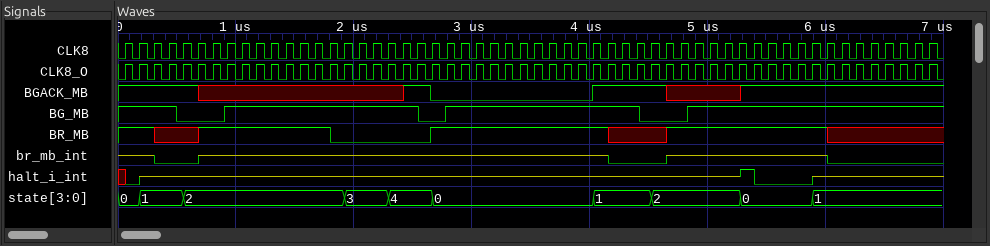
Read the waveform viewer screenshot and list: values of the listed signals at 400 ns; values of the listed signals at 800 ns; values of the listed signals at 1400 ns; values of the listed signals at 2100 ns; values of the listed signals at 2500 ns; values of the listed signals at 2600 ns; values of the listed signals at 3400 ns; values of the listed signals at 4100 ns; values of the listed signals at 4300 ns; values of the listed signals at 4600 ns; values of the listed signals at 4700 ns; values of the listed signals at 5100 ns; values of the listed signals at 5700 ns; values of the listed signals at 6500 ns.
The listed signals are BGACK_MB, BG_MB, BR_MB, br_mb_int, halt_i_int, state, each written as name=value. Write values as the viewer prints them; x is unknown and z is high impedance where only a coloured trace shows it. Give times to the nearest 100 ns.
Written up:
BGACK_MB=1, BG_MB=1, BR_MB=x, br_mb_int=0, halt_i_int=z, state=1
BGACK_MB=x, BG_MB=0, BR_MB=1, br_mb_int=z, halt_i_int=z, state=2
BGACK_MB=x, BG_MB=1, BR_MB=1, br_mb_int=z, halt_i_int=z, state=2
BGACK_MB=x, BG_MB=1, BR_MB=0, br_mb_int=z, halt_i_int=z, state=3
BGACK_MB=1, BG_MB=1, BR_MB=0, br_mb_int=z, halt_i_int=z, state=4
BGACK_MB=1, BG_MB=0, BR_MB=0, br_mb_int=z, halt_i_int=z, state=4
BGACK_MB=0, BG_MB=1, BR_MB=1, br_mb_int=z, halt_i_int=z, state=0
BGACK_MB=1, BG_MB=1, BR_MB=1, br_mb_int=z, halt_i_int=z, state=1
BGACK_MB=1, BG_MB=1, BR_MB=x, br_mb_int=0, halt_i_int=z, state=1
BGACK_MB=1, BG_MB=0, BR_MB=x, br_mb_int=0, halt_i_int=z, state=2
BGACK_MB=x, BG_MB=0, BR_MB=1, br_mb_int=z, halt_i_int=z, state=2
BGACK_MB=x, BG_MB=1, BR_MB=1, br_mb_int=z, halt_i_int=z, state=2
BGACK_MB=1, BG_MB=1, BR_MB=1, br_mb_int=z, halt_i_int=0, state=0
BGACK_MB=1, BG_MB=1, BR_MB=x, br_mb_int=0, halt_i_int=z, state=1
